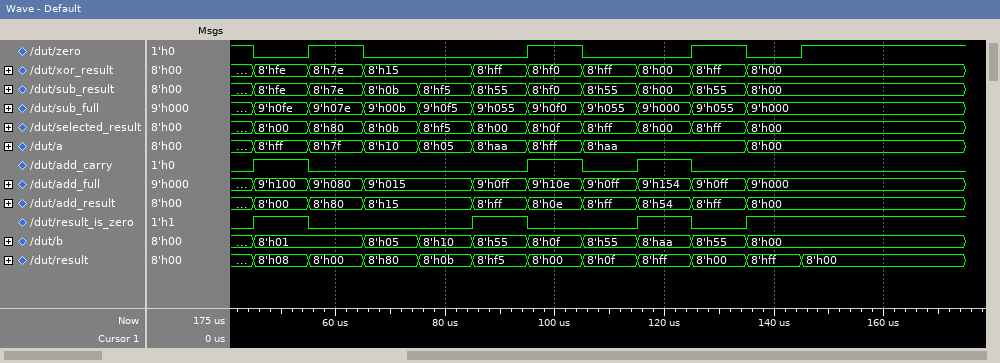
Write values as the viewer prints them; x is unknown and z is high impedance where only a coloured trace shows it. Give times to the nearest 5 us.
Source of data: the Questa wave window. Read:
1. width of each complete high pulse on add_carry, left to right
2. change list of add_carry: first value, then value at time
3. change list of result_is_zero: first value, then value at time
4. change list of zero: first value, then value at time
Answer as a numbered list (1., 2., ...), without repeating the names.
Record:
1. 10 us, 10 us, 10 us
2. 0, 1 at 45 us, 0 at 55 us, 1 at 95 us, 0 at 105 us, 1 at 115 us, 0 at 125 us
3. 0, 1 at 45 us, 0 at 55 us, 1 at 85 us, 0 at 95 us, 1 at 115 us, 0 at 125 us, 1 at 135 us
4. 1, 0 at 45 us, 1 at 55 us, 0 at 65 us, 1 at 95 us, 0 at 105 us, 1 at 125 us, 0 at 135 us, 1 at 145 us
